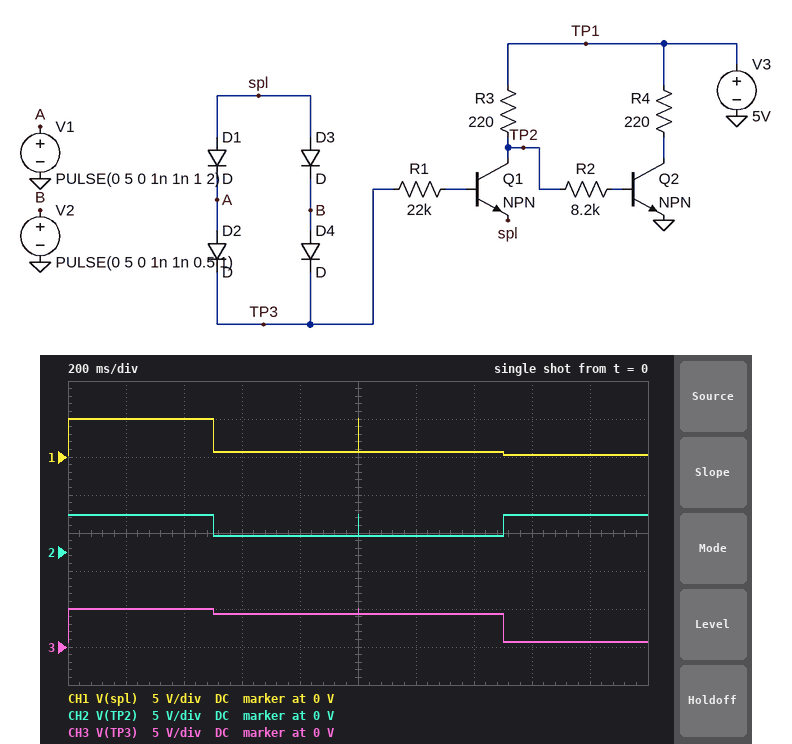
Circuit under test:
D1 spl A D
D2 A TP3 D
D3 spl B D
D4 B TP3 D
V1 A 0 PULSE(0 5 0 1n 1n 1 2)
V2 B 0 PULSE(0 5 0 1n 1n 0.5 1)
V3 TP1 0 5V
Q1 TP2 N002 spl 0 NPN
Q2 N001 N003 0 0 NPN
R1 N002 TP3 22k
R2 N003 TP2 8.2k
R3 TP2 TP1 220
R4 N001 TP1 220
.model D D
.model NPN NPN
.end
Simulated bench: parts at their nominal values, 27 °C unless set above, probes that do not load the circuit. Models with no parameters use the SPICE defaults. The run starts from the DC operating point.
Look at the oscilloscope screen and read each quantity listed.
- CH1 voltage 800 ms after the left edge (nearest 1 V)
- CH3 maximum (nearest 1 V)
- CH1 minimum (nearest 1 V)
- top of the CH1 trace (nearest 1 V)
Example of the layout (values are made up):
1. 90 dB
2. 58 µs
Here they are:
1. 1 V
2. 5 V
3. 0 V
4. 5 V
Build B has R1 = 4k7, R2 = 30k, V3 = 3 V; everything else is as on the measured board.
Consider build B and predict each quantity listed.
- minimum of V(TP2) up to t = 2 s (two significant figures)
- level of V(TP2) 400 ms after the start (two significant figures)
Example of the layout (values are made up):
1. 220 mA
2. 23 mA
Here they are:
1. 800 mV
2. 3.0 V
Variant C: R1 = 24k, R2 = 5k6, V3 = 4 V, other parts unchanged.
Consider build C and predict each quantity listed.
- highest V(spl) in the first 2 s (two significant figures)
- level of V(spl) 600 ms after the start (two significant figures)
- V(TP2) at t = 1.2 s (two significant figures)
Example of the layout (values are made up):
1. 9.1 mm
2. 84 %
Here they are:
1. 3.9 V
2. 720 mV
3. 1.4 V
